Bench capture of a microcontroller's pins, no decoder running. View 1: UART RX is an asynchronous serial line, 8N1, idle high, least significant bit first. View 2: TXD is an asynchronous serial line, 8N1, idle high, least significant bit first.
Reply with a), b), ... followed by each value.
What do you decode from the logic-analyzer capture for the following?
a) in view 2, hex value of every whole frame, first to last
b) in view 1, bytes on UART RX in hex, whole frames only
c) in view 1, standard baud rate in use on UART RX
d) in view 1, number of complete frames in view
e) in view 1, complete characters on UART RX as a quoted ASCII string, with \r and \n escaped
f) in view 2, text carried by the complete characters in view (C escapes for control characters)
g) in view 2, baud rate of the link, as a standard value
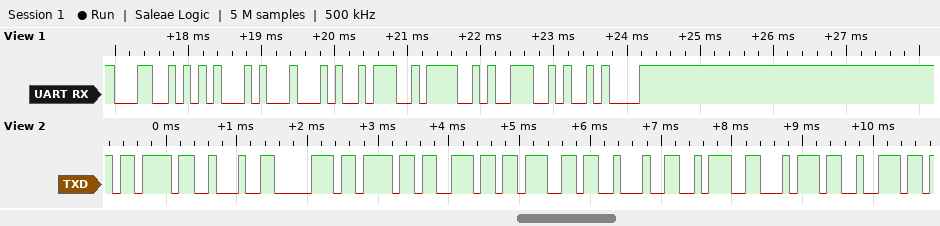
a) 0x7B 0x22 0x70 0x6F 0x6E 0x67 0x22 0x3A 0x74 0x72
b) 4C 45 44 3A 4F 4E 0A
c) 9600 baud
d) 7
e) "LED:ON\n"
f) "{\"pong\":tr"
g) 9600 baud
